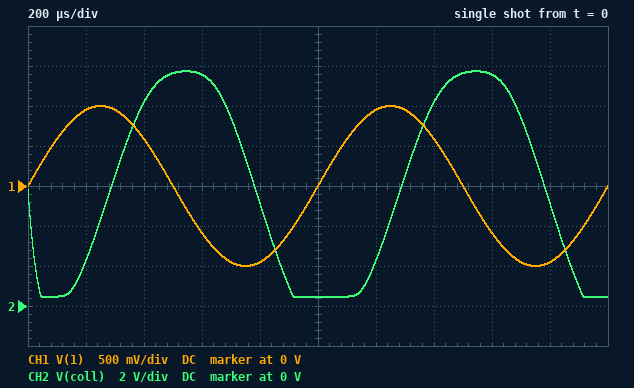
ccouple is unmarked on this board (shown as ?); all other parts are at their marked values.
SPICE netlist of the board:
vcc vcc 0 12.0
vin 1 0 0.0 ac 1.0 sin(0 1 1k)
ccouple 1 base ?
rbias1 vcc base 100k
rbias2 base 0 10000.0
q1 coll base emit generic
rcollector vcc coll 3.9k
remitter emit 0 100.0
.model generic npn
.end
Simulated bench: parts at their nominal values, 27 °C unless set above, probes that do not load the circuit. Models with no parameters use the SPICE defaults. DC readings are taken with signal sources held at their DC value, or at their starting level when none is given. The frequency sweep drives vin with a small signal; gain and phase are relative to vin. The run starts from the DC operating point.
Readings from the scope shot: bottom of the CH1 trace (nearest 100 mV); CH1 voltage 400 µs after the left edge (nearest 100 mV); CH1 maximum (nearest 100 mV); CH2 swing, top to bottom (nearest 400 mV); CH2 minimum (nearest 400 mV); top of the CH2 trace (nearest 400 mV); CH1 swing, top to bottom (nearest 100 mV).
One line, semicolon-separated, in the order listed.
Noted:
-1.0 V; 600 mV; 1.0 V; 11.2 V; 400 mV; 11.6 V; 2.0 V
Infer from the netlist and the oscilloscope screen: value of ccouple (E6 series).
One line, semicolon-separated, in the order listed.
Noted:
6.8 nF
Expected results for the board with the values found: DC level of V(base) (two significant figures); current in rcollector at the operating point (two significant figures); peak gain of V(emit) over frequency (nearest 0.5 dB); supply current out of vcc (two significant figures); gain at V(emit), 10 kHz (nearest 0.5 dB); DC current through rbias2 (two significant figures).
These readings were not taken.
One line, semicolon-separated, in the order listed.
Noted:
950 mV; 1.6 mA; -1.5 dB; 1.7 mA; -2.0 dB; 95 µA
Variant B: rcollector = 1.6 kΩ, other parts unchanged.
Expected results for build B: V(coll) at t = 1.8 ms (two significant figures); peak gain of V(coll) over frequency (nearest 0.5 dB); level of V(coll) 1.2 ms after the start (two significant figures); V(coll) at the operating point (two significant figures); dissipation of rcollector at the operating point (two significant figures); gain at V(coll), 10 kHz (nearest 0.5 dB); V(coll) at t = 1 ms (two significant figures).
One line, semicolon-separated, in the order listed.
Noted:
9.2 V; 22.5 dB; 8.0 V; 9.5 V; 4.0 mW; 22.0 dB; 6.5 V
